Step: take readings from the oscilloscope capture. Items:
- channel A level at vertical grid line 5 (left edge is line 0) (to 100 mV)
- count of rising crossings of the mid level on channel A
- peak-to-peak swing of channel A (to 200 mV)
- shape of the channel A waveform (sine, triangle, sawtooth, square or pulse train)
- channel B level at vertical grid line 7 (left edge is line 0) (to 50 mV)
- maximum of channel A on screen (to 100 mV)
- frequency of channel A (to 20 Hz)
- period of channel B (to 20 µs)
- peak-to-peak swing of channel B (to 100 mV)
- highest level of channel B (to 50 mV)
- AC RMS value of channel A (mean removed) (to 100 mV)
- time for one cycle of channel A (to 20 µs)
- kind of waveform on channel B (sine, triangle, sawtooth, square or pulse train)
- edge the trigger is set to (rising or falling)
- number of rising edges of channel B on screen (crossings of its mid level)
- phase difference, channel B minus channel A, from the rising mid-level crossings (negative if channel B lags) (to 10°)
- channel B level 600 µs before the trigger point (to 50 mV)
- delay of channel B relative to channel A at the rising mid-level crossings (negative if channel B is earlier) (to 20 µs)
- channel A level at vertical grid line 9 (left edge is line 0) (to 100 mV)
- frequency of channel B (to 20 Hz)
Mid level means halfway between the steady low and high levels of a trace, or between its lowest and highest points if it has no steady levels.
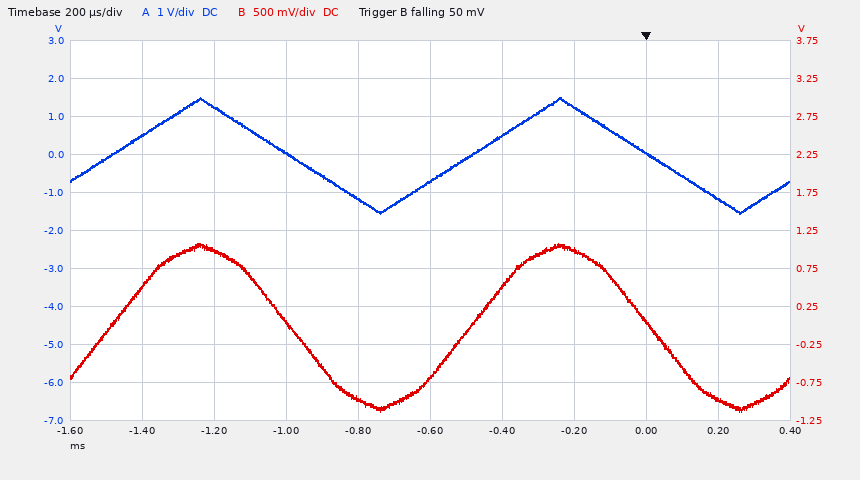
-700 mV
2
3.0 V
triangle
1.00 V
1.5 V
1.00 kHz
1.00 ms
2.20 V
1.10 V
900 mV
1.00 ms
sine
falling
2
0°
-700 mV
0 µs
-1.2 V
1.00 kHz
